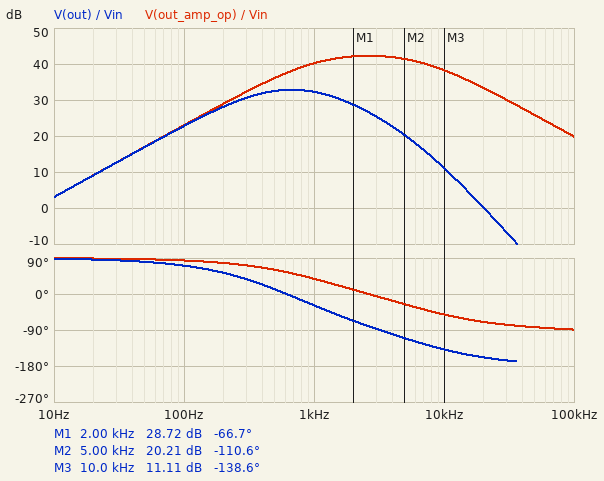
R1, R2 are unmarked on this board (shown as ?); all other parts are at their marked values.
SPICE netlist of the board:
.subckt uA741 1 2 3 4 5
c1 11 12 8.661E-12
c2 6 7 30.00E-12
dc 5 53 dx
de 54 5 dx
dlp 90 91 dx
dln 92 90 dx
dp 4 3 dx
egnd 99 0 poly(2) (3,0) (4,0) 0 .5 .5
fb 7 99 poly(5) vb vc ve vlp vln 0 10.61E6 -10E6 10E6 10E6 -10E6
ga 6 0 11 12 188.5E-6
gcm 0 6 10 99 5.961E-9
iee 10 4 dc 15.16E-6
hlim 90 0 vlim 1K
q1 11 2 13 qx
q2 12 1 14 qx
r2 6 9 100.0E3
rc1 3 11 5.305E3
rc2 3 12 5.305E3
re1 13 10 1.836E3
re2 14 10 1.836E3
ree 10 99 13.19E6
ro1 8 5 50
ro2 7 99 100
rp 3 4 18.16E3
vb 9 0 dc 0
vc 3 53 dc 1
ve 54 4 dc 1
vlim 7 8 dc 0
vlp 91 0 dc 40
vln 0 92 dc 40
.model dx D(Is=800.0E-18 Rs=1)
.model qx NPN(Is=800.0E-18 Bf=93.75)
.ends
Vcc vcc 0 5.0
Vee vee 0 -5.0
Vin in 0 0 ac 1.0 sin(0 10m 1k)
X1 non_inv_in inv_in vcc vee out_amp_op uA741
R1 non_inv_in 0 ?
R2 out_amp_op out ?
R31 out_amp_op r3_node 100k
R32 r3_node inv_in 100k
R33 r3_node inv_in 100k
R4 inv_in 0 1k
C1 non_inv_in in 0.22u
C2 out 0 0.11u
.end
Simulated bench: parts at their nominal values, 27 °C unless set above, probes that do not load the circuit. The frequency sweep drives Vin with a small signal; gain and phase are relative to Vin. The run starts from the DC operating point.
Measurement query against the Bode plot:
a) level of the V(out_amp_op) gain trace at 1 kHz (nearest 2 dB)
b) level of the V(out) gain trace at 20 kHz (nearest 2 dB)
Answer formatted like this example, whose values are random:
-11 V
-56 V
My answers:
40 dB
0 dB
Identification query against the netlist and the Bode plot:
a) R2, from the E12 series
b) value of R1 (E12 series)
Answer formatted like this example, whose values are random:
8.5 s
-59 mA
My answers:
3.3 kΩ
680 Ω
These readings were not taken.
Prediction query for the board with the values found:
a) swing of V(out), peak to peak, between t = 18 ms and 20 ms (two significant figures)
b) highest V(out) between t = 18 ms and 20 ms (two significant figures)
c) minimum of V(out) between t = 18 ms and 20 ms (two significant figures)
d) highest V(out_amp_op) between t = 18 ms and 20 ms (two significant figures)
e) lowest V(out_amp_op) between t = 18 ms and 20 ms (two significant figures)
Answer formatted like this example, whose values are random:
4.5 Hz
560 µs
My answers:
820 mV
420 mV
-400 mV
1.0 V
-1.0 V
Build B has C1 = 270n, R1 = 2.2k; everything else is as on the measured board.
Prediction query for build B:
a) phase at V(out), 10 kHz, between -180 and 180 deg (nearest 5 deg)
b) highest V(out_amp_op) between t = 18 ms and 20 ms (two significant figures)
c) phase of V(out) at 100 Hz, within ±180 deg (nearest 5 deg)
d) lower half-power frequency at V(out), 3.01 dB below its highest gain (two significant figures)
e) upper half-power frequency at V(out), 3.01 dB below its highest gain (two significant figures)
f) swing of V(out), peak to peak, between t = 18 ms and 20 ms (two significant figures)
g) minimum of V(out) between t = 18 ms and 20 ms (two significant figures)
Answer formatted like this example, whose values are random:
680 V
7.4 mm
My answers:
-145 deg
1.4 V
55 deg
140 Hz
840 Hz
1.2 V
-590 mV
